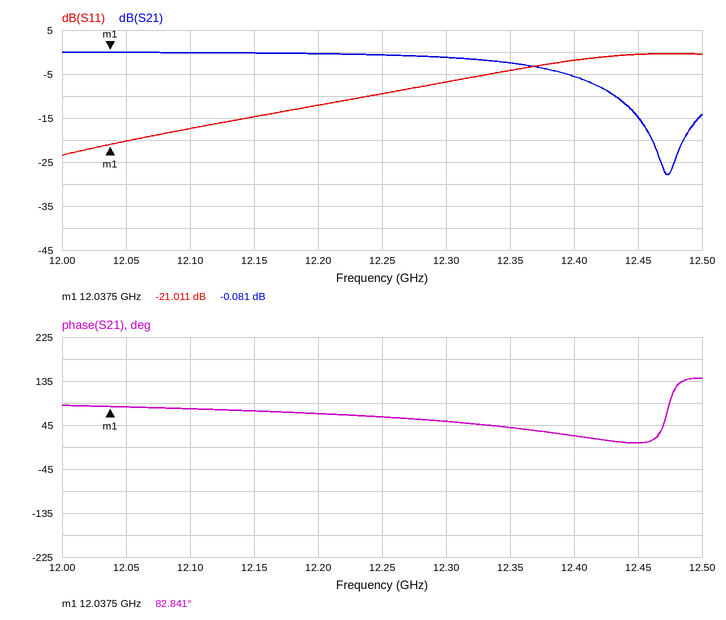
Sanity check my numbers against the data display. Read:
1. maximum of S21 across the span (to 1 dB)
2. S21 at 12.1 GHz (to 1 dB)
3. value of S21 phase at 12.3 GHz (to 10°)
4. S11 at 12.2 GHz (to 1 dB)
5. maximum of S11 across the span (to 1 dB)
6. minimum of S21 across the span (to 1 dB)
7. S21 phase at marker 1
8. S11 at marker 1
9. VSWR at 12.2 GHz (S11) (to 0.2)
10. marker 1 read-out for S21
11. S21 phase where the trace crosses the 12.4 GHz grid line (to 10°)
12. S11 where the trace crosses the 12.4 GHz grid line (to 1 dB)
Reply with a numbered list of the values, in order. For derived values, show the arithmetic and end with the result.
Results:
1. 0 dB
2. 0 dB
3. 50°
4. -12 dB
5. 0 dB
6. -28 dB
7. 82.841°
8. -21.011 dB
9. |Γ| = 10^(-12/20) = 0.2512; VSWR = (1 + 0.2512)/(1 − 0.2512) ≈ 1.67, so 1.6 to the nearest 0.2
10. -0.081 dB
11. 20°
12. -2 dB
